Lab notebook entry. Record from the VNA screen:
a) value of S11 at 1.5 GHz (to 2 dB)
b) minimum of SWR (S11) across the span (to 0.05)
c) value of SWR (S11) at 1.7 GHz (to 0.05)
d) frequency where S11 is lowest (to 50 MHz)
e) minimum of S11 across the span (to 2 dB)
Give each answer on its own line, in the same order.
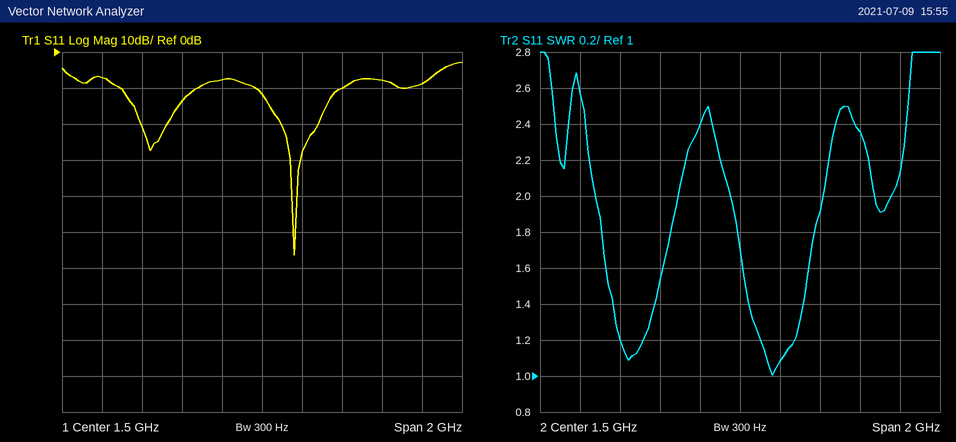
-12 dB
1.00
1.10
1.65 GHz
-56 dB
